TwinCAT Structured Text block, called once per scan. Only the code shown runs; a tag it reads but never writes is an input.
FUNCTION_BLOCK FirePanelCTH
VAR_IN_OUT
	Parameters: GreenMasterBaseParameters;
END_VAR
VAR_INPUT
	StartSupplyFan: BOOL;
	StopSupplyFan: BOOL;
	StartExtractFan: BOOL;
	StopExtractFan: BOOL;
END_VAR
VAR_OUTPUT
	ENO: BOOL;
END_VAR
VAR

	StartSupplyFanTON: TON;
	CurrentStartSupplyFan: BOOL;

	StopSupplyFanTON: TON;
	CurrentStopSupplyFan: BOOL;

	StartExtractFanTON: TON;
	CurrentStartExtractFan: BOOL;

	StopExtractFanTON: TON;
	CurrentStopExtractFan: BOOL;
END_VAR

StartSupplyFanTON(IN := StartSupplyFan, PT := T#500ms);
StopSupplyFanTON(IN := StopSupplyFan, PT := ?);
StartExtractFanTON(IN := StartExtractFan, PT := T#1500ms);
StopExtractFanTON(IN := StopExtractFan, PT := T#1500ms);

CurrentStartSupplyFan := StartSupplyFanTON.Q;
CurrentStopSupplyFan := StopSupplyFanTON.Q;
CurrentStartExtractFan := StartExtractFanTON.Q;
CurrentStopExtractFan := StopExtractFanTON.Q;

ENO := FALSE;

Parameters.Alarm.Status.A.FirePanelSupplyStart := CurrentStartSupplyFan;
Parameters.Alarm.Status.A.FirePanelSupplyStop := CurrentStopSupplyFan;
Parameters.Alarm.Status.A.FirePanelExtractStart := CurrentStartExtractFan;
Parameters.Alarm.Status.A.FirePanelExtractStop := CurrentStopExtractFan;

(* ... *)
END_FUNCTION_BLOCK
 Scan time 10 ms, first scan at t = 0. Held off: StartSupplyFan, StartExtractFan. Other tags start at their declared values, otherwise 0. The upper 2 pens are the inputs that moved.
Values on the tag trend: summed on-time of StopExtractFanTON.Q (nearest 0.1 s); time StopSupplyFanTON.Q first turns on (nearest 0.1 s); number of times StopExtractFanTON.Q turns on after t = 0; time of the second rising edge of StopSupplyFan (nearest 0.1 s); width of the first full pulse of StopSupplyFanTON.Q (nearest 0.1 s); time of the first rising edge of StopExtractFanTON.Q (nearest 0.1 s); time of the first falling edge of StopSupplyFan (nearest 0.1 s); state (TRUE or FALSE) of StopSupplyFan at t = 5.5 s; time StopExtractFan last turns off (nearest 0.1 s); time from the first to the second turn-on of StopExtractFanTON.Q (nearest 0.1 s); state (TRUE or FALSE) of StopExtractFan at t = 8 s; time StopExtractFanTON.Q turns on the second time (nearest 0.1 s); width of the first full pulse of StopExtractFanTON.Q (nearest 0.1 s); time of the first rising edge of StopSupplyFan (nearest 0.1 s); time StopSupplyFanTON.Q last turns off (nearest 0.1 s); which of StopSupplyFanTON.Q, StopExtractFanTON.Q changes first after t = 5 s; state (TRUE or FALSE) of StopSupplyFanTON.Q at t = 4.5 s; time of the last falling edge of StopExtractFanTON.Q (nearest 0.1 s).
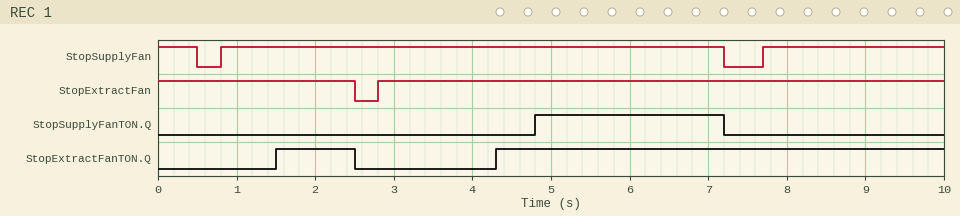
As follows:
6.7 s
4.8 s
2
7.7 s
2.4 s
1.5 s
0.5 s
TRUE
2.5 s
2.8 s
TRUE
4.3 s
1.0 s
0.8 s
7.2 s
StopSupplyFanTON.Q
FALSE
2.5 s
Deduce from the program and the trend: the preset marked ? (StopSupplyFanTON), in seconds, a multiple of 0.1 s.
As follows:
4.0 s
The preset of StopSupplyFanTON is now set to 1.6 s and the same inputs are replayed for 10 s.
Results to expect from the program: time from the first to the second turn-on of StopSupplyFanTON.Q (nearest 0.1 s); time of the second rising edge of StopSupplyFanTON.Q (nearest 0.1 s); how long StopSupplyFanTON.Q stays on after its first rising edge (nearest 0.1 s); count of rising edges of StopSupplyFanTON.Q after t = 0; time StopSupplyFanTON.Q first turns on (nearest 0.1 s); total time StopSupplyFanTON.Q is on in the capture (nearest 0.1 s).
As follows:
6.9 s
9.3 s
4.8 s
2
2.4 s
5.5 s
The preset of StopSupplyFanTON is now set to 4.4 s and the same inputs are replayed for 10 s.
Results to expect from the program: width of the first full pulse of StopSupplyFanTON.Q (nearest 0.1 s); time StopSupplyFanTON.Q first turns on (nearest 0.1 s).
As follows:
2.0 s
5.2 s
